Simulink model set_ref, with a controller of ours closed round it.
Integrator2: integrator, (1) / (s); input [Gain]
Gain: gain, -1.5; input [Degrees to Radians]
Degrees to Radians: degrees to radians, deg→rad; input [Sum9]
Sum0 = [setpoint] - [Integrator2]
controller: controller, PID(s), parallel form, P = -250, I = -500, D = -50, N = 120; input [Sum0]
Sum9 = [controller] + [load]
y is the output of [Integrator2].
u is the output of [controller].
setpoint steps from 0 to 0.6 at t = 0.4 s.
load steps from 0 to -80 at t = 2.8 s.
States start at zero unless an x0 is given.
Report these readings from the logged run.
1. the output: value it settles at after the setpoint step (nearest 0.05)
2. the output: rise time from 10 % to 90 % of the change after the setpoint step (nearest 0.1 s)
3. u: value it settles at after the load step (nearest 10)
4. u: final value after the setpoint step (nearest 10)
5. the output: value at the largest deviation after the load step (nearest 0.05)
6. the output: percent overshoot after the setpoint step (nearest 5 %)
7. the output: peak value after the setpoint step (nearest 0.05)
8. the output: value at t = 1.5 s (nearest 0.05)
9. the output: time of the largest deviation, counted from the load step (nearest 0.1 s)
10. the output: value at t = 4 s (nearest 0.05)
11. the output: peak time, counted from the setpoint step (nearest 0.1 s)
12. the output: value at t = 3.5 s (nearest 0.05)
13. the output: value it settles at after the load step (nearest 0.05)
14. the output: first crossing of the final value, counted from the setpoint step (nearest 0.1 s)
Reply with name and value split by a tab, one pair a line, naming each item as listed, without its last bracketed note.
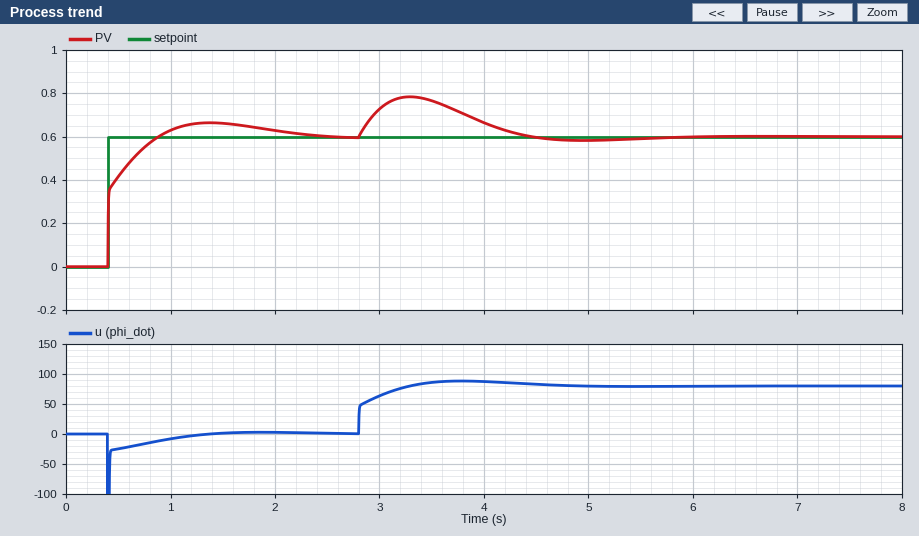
the output: value it settles at after the setpoint step	0.60
the output: rise time from 10 % to 90 % of the change after the setpoint step	0.3 s
u: value it settles at after the load step	80
u: final value after the setpoint step	0
the output: value at the largest deviation after the load step	0.80
the output: percent overshoot after the setpoint step	10 %
the output: peak value after the setpoint step	0.65
the output: value at t = 1.5 s	0.65
the output: time of the largest deviation, counted from the load step	0.5 s
the output: value at t = 4 s	0.65
the output: peak time, counted from the setpoint step	1.0 s
the output: value at t = 3.5 s	0.75
the output: value it settles at after the load step	0.60
the output: first crossing of the final value, counted from the setpoint step	0.5 s
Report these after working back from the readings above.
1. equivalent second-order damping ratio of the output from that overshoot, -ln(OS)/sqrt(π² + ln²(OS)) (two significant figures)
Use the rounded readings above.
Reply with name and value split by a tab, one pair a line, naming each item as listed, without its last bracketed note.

equivalent second-order damping ratio of the output from that overshoot, -ln(OS)/sqrt(π² + ln²(OS))	0.59
